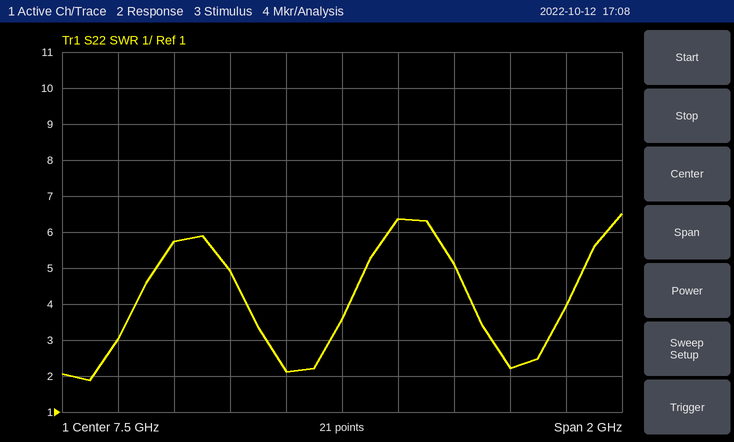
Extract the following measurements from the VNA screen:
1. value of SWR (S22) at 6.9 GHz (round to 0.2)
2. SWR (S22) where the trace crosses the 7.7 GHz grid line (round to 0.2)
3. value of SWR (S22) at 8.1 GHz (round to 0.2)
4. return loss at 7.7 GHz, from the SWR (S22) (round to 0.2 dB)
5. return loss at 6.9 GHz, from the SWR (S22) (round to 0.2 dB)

5.8
6.4
2.2
2.8 dB
3.0 dB
